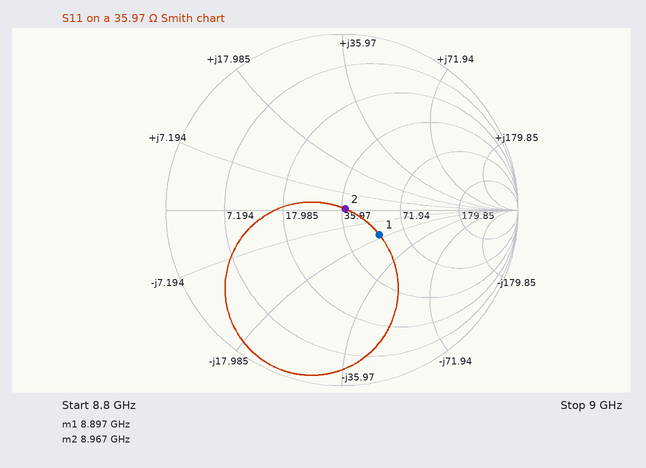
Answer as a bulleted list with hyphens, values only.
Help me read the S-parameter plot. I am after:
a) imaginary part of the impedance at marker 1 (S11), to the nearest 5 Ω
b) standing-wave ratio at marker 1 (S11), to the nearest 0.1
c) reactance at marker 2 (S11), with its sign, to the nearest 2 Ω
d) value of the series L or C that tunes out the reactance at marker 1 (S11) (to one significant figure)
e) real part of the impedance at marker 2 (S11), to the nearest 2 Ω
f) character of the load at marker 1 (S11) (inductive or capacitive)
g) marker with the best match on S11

- -15 Ω
- 1.7
- 0 Ω
- 300 pH
- 38 Ω
- capacitive
- marker 2
